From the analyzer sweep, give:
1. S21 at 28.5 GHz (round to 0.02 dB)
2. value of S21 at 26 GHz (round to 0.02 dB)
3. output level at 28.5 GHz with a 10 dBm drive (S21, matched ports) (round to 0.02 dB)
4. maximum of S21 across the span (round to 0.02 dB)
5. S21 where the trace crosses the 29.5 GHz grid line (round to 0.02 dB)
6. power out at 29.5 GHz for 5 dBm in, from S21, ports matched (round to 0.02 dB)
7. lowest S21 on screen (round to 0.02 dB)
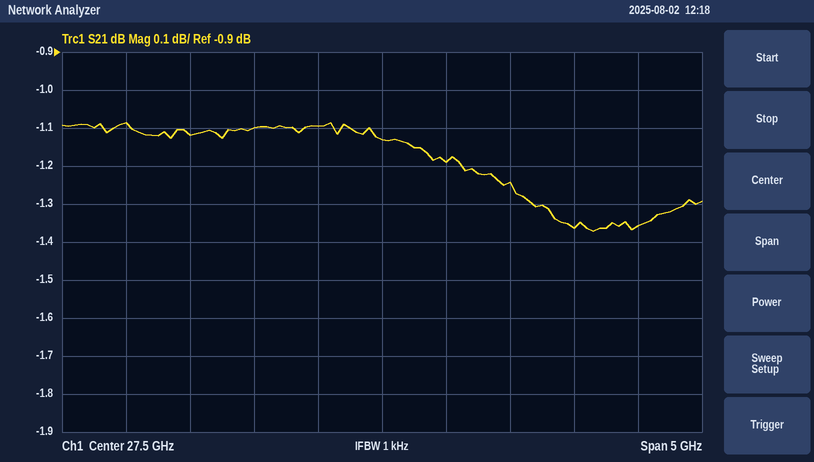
-1.24 dB
-1.12 dB
8.76 dBm
-1.08 dB
-1.36 dB
3.64 dBm
-1.38 dB
